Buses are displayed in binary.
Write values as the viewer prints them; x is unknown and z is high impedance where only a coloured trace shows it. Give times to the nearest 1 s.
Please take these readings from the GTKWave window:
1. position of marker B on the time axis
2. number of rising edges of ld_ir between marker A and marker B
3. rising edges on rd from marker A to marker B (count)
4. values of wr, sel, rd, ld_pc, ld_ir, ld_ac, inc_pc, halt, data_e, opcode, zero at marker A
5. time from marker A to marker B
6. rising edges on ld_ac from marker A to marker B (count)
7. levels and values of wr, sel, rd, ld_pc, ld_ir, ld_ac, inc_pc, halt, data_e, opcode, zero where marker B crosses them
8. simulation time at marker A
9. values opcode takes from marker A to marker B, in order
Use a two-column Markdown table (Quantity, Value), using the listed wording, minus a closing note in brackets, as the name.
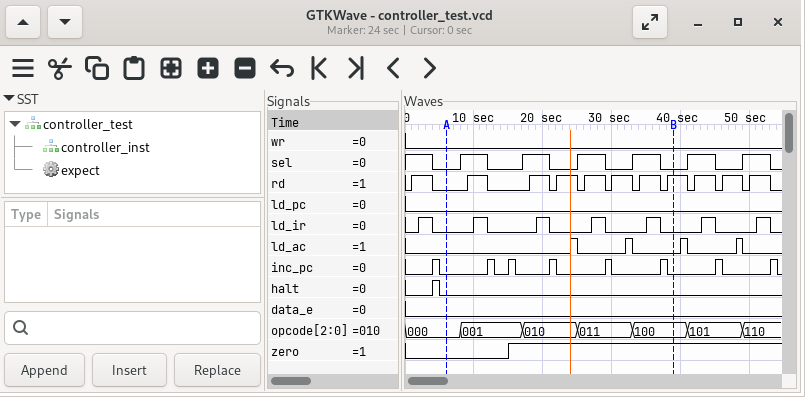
| Quantity | Value |
|---|---|
| position of marker B on the time axis | 39 s |
| number of rising edges of ld_ir between marker A and marker B | 4 |
| rising edges on rd from marker A to marker B | 7 |
| values of wr, sel, rd, ld_pc, ld_ir, ld_ac, inc_pc, halt, data_e, opcode, zero at marker A | wr=0, sel=0, rd=0, ld_pc=0, ld_ir=0, ld_ac=0, inc_pc=0, halt=0, data_e=0, opcode=000, zero=0 |
| time from marker A to marker B | 33 s |
| rising edges on ld_ac from marker A to marker B | 2 |
| levels and values of wr, sel, rd, ld_pc, ld_ir, ld_ac, inc_pc, halt, data_e, opcode, zero where marker B crosses them | wr=0, sel=0, rd=1, ld_pc=0, ld_ir=0, ld_ac=0, inc_pc=0, halt=0, data_e=0, opcode=100, zero=1 |
| simulation time at marker A | 6 s |
| values opcode takes from marker A to marker B, in order | 000, 001, 010, 011, 100 |
